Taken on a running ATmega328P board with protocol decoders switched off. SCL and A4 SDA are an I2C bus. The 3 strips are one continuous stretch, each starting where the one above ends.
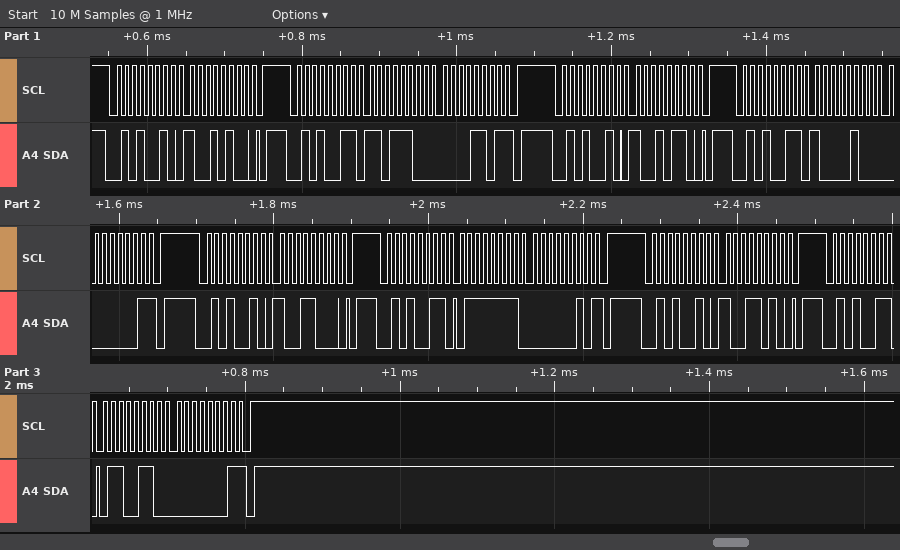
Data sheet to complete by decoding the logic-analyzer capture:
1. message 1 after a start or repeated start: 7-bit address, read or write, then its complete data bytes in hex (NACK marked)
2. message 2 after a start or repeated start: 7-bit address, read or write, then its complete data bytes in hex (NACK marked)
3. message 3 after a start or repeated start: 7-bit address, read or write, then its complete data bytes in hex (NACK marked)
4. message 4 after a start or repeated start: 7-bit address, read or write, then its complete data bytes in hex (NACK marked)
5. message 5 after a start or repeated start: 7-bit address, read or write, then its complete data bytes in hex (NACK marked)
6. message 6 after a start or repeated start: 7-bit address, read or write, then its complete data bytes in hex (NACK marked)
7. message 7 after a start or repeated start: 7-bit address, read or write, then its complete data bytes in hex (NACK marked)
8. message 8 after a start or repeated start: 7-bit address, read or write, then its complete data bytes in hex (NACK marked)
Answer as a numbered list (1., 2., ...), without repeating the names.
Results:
1. 0x29 write: 94
2. 0x29 read: DC 0D NACK
3. 0x29 write: 96
4. 0x29 read: 84 01 NACK
5. 0x29 write: 98
6. 0x29 read: 7F 02 NACK
7. 0x29 write: 9A
8. 0x29 read: 66 01 NACK
